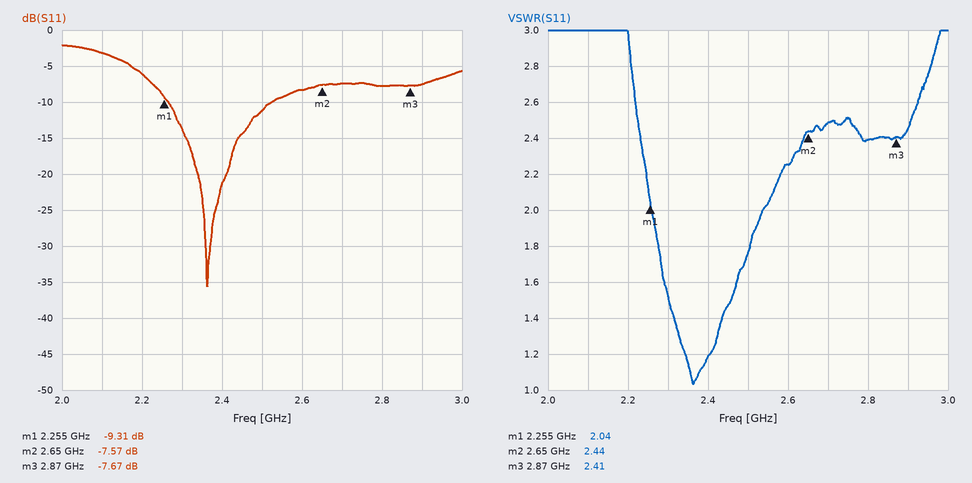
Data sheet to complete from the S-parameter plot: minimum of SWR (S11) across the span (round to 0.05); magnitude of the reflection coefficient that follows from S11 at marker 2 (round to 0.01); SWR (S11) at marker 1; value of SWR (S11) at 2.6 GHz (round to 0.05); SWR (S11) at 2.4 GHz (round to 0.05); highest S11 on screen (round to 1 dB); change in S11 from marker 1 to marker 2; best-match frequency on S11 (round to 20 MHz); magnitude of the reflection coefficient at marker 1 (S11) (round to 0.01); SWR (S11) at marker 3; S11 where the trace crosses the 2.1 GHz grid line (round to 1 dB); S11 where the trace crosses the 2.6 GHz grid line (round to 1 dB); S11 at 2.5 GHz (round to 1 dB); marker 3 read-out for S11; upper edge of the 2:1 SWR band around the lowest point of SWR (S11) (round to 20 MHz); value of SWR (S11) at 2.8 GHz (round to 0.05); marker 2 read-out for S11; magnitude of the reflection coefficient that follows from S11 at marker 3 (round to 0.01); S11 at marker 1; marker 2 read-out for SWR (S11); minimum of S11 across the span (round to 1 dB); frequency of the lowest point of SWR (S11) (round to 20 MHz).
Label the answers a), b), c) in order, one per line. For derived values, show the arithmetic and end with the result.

a) 1.05
b) 10^(-7.57/20) ≈ 0.42
c) 2.04
d) 2.25
e) 1.20
f) -2 dB
g) -7.57 − (-9.31) = 1.74 dB
h) 2.36 GHz
i) 10^(-9.31/20) ≈ 0.34
j) 2.41
k) -3 dB
l) -8 dB
m) -11 dB
n) -7.67 dB
o) 2.54 GHz
p) 2.40
q) -7.57 dB
r) 10^(-7.67/20) ≈ 0.41
s) -9.31 dB
t) 2.44
u) -36 dB
v) 2.36 GHz
